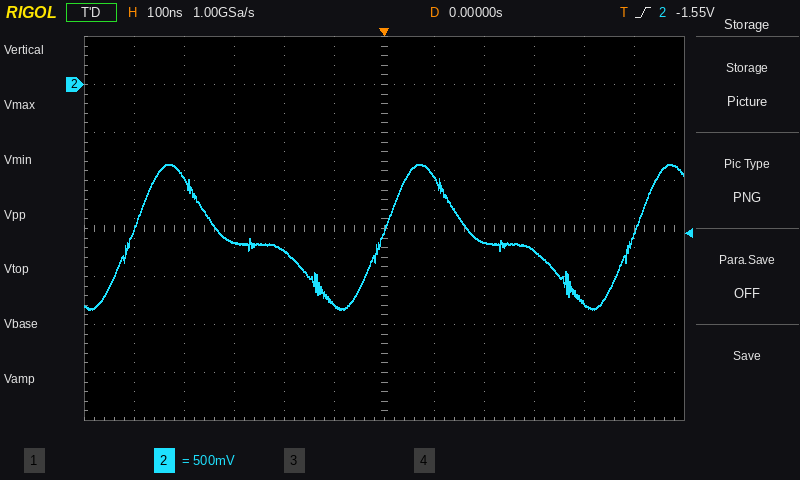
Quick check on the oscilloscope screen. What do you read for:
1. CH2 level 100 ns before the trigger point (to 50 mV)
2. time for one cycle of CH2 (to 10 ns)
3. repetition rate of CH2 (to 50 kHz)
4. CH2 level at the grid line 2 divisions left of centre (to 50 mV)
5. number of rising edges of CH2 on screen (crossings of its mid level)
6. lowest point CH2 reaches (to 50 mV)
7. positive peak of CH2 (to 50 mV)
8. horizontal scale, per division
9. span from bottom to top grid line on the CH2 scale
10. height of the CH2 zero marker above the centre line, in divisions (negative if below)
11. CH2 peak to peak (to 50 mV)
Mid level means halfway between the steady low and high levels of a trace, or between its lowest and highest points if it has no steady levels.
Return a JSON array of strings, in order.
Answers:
["-2.30 V", "500 ns", "2.00 MHz", "-1.75 V", "3", "-2.35 V", "-850 mV", "100 ns", "4 V", "+3.0 div", "1.50 V"]
